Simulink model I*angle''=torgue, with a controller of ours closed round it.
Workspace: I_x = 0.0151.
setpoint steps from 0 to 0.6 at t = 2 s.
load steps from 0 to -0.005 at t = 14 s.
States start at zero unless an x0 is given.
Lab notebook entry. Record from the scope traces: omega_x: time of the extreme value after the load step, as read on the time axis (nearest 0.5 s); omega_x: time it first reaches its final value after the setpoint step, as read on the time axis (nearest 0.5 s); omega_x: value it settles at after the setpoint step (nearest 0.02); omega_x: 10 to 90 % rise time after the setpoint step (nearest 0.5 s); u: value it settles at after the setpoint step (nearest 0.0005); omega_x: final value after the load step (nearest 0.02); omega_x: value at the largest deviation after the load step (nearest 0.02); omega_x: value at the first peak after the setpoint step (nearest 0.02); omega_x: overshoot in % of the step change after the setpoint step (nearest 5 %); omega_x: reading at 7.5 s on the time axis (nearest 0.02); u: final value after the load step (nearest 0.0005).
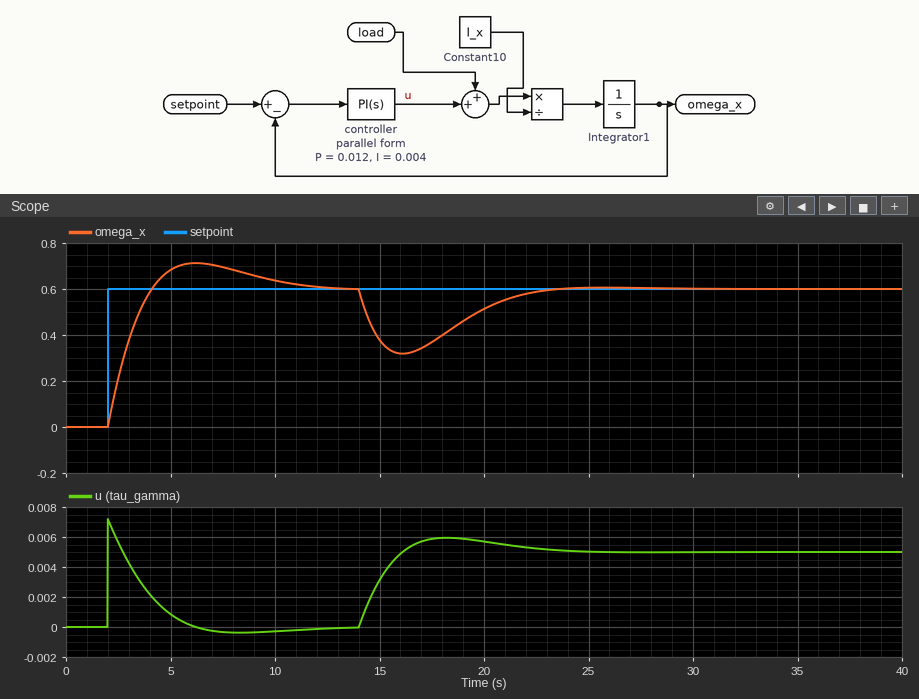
16.0 s
4.0 s
0.60
1.5 s
0.0000
0.60
0.32
0.72
20 %
0.70
0.0050
